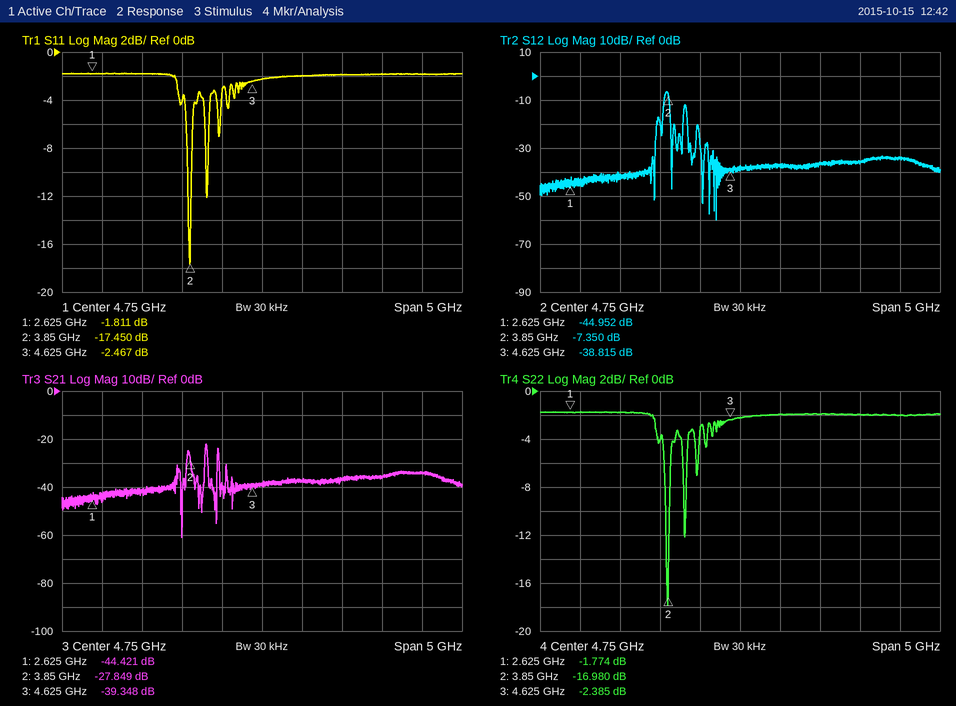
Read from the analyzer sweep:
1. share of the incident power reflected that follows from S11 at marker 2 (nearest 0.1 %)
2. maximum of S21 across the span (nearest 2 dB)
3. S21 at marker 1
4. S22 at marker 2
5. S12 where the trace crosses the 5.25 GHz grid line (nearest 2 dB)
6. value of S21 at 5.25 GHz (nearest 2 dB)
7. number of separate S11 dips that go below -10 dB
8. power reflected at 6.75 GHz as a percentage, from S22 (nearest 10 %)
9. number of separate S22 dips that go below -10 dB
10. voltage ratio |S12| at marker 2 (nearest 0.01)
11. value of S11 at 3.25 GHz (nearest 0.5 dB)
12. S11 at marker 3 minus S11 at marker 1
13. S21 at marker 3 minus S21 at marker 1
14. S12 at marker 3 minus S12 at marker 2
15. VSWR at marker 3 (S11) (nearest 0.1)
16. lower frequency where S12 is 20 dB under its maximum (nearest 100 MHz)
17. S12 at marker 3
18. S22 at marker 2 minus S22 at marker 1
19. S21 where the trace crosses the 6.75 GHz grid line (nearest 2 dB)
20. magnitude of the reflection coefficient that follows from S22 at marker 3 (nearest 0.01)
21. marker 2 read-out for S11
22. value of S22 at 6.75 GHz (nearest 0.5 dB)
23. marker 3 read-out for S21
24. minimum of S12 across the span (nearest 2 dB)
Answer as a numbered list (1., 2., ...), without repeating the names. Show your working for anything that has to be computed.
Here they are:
1. 10^(-17.45/10) ≈ 1.8 %
2. -22 dB
3. -44.421 dB
4. -16.980 dB
5. -38 dB
6. -38 dB
7. 2
8. 10^(-2/10) ≈ 63.1 %, so 60 % to the nearest 10 %
9. 2
10. 10^(-7.35/20) ≈ 0.43
11. -2.0 dB
12. -2.467 − (-1.811) = -0.656 dB
13. -39.348 − (-44.421) = 5.073 dB
14. -38.815 − (-7.35) = -31.465 dB
15. (1 + 0.7527)/(1 − 0.7527) ≈ 7.1
16. 3.7 GHz
17. -38.815 dB
18. -16.98 − (-1.774) = -15.206 dB
19. -34 dB
20. 10^(-2.385/20) ≈ 0.76
21. -17.450 dB
22. -2.0 dB
23. -39.348 dB
24. -60 dB
